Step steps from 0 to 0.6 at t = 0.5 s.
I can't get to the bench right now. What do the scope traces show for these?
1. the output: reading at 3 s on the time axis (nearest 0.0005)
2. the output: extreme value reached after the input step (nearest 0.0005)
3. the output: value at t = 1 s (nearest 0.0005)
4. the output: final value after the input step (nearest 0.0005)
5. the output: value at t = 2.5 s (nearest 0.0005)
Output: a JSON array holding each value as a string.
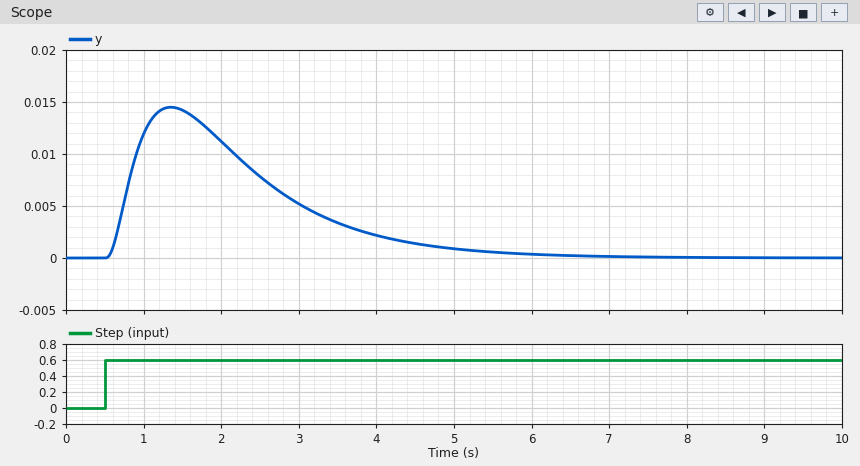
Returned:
["0.0050", "0.0145", "0.0120", "0.0000", "0.0080"]
